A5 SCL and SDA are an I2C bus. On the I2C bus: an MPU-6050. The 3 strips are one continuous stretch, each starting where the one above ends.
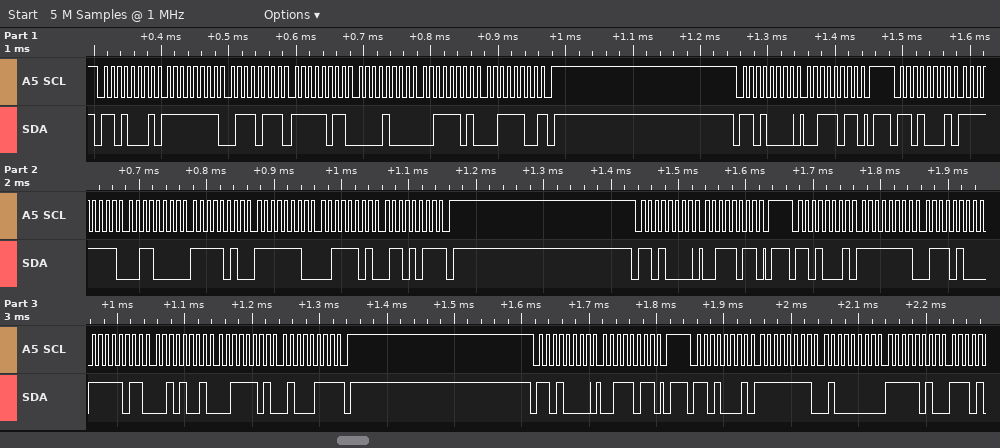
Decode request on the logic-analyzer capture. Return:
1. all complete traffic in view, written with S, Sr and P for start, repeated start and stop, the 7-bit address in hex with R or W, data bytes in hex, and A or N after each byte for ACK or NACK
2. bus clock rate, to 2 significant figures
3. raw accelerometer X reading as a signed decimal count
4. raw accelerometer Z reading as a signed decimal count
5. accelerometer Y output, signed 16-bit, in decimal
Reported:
S 68R A FF A 77 A FB A 08 A 3D A 3C N P S 68W A 3B A P S 68R A FF A 30 A FA A FE A 3D A 6B N P S 68W A 3B A P S 68R A FF A 74 A FB A 29 A 3D A 47 N P S 68W A 3B A P S 68R A FF A 40 A FA A
100 kHz
-208
15723
-1282
